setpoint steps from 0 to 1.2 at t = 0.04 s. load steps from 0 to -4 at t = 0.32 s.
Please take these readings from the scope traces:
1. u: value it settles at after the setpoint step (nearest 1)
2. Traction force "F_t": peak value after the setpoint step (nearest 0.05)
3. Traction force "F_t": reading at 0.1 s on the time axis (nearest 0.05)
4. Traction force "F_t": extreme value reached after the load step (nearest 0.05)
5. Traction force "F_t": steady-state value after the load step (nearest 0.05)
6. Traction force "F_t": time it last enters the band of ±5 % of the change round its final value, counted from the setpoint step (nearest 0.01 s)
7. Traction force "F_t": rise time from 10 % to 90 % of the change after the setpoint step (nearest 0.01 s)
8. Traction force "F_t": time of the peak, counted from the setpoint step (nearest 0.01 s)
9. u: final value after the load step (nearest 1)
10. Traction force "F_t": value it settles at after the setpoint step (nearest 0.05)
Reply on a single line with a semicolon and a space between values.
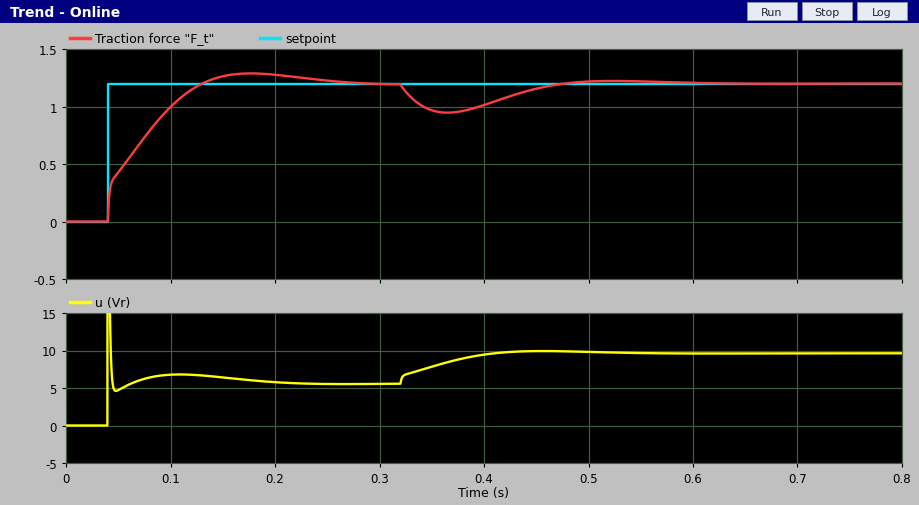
6; 1.30; 1.00; 0.95; 1.20; 0.18 s; 0.07 s; 0.14 s; 10; 1.20
